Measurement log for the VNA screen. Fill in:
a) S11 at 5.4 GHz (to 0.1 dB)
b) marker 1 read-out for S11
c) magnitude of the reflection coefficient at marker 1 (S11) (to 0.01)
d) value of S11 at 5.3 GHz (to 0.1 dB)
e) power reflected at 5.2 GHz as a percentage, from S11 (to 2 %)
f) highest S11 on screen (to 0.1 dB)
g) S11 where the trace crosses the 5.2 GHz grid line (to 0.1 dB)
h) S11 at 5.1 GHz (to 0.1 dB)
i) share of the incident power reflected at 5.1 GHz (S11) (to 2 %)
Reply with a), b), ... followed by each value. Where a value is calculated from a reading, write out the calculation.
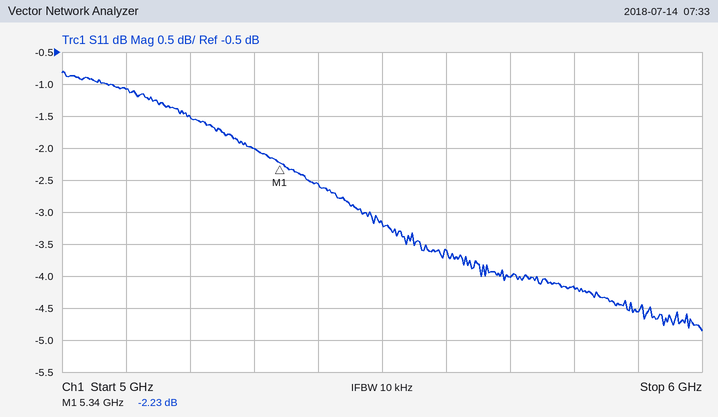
a) -2.6 dB
b) -2.23 dB
c) 10^(-2.23/20) ≈ 0.77
d) -2.0 dB
e) 10^(-1.5/10) ≈ 70.8 %, so 70 % to the nearest 2 %
f) -0.8 dB
g) -1.5 dB
h) -1.1 dB
i) 10^(-1.1/10) ≈ 78 %
